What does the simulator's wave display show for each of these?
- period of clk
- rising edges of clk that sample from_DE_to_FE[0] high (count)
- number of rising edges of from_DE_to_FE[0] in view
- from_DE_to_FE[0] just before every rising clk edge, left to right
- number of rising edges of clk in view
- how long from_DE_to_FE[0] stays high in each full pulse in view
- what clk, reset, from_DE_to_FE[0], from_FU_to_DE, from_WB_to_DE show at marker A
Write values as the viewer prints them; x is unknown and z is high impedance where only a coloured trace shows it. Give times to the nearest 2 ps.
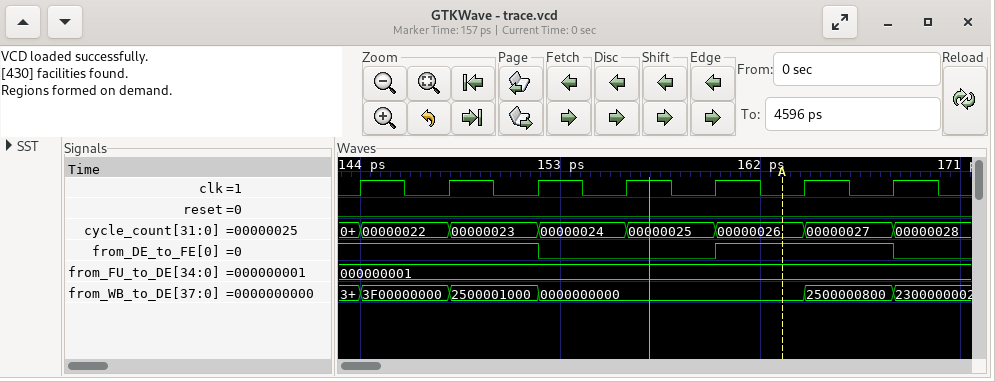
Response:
4 ps
5
1
1 1 1 0 0 1 1
7
8 ps
clk=0, reset=0, from_DE_to_FE[0]=1, from_FU_to_DE=000000001, from_WB_to_DE=0000000000
